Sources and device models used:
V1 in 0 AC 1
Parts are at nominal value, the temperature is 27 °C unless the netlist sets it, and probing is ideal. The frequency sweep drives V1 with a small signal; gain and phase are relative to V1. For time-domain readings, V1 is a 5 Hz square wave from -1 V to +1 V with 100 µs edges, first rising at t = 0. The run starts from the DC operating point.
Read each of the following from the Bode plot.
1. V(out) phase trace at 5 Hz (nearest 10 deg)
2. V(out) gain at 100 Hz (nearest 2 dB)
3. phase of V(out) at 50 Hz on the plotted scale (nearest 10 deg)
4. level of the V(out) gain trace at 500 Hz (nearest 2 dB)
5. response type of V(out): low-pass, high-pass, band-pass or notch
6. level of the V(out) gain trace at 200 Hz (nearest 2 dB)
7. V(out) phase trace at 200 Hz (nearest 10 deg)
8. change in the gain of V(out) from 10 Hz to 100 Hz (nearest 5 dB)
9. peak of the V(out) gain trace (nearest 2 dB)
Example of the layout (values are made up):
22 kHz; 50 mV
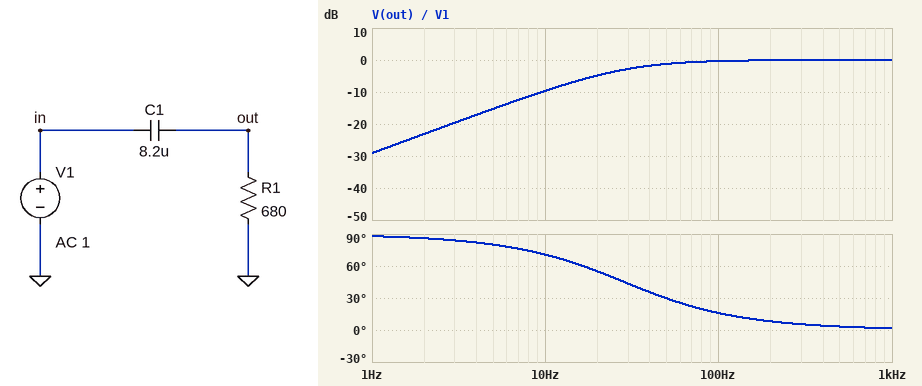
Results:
80 deg; 0 dB; 30 deg; 0 dB; high-pass; 0 dB; 10 deg; 10 dB; 0 dB
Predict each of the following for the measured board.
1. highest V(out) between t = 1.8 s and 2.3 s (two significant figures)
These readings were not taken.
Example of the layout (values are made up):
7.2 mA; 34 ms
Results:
2.0 V
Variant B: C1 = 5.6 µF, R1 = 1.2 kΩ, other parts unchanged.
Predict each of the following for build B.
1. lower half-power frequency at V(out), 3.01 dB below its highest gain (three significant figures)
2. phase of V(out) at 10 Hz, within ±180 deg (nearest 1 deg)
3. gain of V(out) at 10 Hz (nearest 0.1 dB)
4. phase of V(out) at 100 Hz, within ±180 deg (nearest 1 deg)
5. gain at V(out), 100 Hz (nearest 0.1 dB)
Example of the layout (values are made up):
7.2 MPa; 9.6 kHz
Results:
23.7 Hz; 67 deg; -8.2 dB; 13 deg; -0.2 dB
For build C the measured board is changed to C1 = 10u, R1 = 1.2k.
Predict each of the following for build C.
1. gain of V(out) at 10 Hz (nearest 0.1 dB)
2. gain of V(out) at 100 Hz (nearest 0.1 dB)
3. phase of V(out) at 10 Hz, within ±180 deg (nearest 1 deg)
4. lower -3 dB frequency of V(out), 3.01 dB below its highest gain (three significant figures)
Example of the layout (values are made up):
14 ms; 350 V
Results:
-4.4 dB; -0.1 dB; 53 deg; 13.3 Hz
